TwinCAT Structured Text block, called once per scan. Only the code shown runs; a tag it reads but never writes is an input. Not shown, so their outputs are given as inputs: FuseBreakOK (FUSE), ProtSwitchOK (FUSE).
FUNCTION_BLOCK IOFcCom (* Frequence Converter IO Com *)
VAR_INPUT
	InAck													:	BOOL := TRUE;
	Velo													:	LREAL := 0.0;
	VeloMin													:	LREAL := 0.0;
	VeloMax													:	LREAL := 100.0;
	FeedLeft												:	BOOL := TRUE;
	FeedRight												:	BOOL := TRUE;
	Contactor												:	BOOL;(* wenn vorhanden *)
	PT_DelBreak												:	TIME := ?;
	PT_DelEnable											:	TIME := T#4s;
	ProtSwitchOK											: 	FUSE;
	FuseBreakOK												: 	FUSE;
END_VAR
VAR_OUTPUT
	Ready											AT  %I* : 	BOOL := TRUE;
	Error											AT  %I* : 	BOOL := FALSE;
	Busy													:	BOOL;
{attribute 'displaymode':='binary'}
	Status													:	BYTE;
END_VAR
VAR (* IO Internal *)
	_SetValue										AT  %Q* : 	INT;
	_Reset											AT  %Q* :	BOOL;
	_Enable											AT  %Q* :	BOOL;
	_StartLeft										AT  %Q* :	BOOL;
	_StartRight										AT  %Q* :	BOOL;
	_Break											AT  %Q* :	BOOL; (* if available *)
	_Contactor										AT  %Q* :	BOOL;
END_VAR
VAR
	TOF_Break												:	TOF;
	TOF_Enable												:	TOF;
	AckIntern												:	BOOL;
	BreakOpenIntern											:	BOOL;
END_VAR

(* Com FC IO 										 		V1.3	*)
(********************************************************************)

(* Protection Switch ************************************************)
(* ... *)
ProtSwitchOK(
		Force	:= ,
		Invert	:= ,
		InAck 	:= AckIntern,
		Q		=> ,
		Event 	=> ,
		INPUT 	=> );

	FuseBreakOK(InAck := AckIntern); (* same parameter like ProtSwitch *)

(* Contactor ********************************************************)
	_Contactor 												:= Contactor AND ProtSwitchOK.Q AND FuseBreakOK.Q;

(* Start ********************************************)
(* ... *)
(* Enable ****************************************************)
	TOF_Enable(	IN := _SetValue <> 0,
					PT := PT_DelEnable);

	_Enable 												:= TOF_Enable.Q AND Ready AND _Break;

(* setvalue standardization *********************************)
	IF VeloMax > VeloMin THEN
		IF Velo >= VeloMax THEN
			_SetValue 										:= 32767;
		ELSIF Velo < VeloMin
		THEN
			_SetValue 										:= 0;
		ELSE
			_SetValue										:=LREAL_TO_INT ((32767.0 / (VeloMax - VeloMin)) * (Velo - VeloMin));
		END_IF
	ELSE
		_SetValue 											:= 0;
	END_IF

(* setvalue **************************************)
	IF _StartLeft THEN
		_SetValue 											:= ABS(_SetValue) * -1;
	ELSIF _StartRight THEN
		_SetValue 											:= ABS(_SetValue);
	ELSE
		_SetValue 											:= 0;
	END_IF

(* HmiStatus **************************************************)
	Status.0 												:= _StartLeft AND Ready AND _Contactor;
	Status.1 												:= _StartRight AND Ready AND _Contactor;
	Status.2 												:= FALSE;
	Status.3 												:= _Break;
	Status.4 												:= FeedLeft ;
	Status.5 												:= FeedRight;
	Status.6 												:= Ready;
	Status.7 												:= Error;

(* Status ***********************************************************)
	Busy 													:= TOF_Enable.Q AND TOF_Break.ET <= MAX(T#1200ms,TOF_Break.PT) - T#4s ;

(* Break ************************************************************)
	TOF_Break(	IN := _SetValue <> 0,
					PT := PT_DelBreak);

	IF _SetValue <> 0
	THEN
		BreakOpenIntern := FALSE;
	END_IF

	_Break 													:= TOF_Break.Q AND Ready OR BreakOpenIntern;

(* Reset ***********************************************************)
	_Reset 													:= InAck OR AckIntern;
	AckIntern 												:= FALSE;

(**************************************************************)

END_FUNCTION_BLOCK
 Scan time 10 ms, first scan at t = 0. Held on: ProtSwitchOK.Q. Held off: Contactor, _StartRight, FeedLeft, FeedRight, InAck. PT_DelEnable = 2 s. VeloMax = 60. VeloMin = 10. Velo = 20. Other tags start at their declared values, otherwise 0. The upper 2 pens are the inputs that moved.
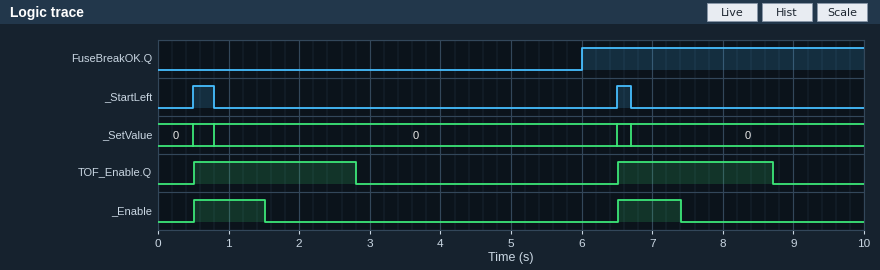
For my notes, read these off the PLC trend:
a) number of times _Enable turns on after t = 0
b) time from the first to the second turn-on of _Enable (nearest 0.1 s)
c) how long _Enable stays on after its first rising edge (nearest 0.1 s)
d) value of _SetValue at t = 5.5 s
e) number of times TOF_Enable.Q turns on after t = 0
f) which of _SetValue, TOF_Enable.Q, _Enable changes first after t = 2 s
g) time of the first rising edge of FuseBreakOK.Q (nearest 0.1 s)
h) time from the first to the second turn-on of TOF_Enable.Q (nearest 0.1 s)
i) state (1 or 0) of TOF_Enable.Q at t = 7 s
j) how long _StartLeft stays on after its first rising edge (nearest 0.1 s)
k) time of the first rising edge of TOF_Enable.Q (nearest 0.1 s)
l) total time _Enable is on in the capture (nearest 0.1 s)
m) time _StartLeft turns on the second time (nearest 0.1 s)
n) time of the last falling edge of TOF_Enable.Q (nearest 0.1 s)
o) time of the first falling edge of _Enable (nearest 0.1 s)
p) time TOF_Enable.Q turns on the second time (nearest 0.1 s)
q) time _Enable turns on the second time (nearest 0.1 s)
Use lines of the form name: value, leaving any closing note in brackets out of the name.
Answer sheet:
number of times _Enable turns on after t = 0: 2
time from the first to the second turn-on of _Enable: 6.0 s
how long _Enable stays on after its first rising edge: 1.0 s
value of _SetValue at t = 5.5 s: 0
number of times TOF_Enable.Q turns on after t = 0: 2
which of _SetValue, TOF_Enable.Q, _Enable changes first after t = 2 s: TOF_Enable.Q
time of the first rising edge of FuseBreakOK.Q: 6.0 s
time from the first to the second turn-on of TOF_Enable.Q: 6.0 s
state (1 or 0) of TOF_Enable.Q at t = 7 s: 1
how long _StartLeft stays on after its first rising edge: 0.3 s
time of the first rising edge of TOF_Enable.Q: 0.5 s
total time _Enable is on in the capture: 1.9 s
time _StartLeft turns on the second time: 6.5 s
time of the last falling edge of TOF_Enable.Q: 8.7 s
time of the first falling edge of _Enable: 1.5 s
time TOF_Enable.Q turns on the second time: 6.5 s
time _Enable turns on the second time: 6.5 s
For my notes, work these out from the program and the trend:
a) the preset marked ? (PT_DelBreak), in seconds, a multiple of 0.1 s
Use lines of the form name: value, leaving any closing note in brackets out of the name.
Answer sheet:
the preset marked ? (PT_DelBreak), in seconds, a multiple of 0.1 s: 0.7 s
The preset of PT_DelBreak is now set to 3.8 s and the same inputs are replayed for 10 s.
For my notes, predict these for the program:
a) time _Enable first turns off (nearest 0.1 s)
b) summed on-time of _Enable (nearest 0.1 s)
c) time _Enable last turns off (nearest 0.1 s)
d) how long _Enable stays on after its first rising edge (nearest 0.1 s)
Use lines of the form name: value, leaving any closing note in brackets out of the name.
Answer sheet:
time _Enable first turns off: 2.8 s
summed on-time of _Enable: 4.5 s
time _Enable last turns off: 8.7 s
how long _Enable stays on after its first rising edge: 2.3 s
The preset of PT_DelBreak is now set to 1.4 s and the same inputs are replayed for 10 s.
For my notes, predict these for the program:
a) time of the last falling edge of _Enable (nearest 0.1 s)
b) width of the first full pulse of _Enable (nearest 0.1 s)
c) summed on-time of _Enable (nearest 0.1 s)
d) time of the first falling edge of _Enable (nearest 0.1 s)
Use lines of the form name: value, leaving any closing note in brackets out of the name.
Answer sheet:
time of the last falling edge of _Enable: 8.1 s
width of the first full pulse of _Enable: 1.7 s
summed on-time of _Enable: 3.3 s
time of the first falling edge of _Enable: 2.2 s
